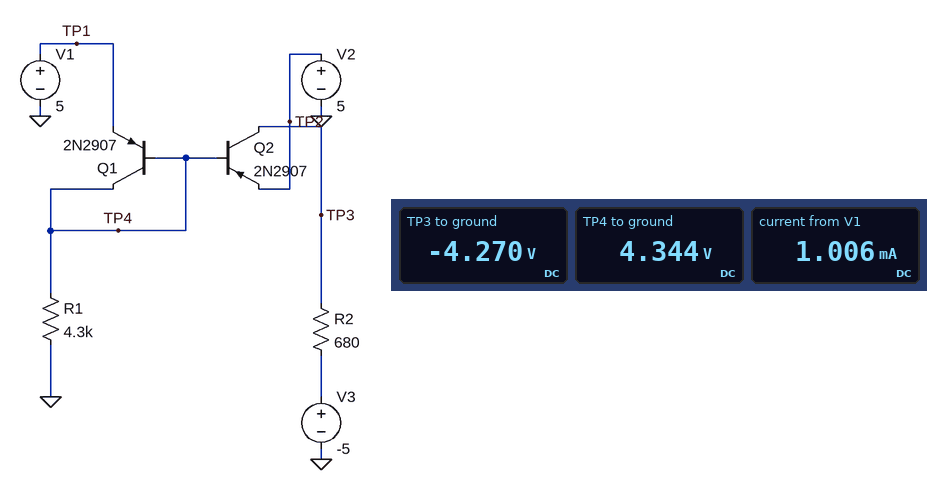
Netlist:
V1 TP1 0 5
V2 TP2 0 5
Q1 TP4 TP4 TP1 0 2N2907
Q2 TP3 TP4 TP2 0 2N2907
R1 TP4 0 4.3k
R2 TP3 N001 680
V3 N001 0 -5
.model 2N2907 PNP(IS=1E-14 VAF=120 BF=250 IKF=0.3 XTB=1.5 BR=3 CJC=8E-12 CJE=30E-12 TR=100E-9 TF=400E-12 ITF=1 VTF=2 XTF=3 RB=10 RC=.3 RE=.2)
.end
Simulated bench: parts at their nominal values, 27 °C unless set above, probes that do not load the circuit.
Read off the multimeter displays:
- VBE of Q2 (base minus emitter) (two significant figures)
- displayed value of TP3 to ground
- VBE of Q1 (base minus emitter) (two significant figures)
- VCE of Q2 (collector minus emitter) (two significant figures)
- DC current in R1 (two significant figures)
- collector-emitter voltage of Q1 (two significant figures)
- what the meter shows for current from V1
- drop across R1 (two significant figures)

-660 mV
-4.270 V
-660 mV
-9.3 V
1.0 mA
-660 mV
1.006 mA
4.3 V
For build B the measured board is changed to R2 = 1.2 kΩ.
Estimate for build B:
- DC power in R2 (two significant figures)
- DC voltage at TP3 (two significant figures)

1.4 mW
-3.7 V
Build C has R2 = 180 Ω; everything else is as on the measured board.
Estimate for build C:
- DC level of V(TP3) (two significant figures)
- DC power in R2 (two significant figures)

-4.8 V
210 µW
